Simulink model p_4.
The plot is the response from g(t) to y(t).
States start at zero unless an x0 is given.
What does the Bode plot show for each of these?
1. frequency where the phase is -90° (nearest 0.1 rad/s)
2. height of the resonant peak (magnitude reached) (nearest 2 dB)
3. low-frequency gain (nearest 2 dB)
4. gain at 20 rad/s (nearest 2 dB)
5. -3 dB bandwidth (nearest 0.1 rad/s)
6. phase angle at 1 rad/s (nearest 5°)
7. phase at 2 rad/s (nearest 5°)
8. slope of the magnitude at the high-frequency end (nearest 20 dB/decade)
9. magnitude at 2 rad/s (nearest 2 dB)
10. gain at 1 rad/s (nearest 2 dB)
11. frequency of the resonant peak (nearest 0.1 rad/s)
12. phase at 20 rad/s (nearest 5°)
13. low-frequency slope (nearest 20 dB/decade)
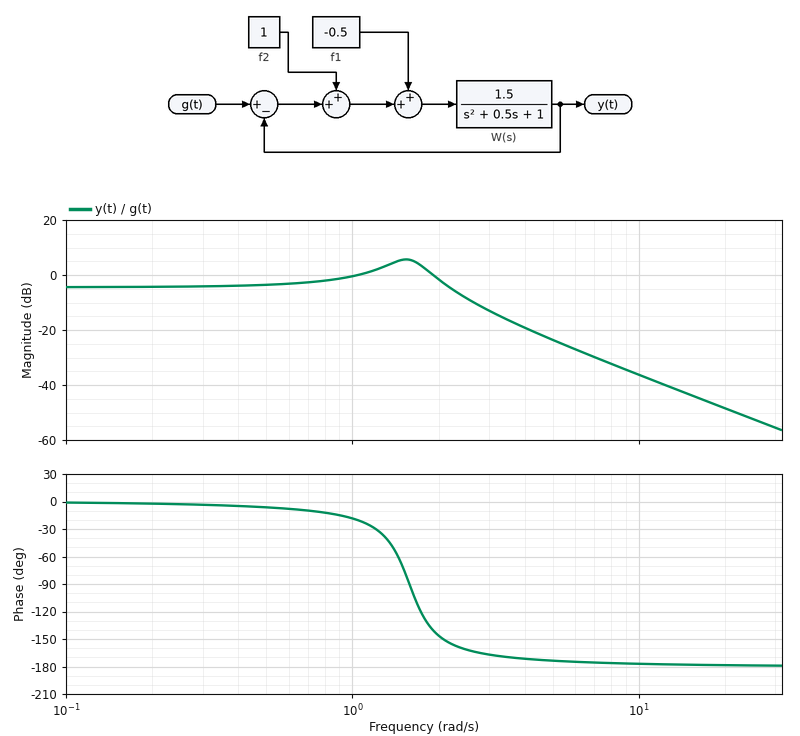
1.6 rad/s
6 dB
-4 dB
-48 dB
2.4 rad/s
-20°
-145°
-40 dB/decade
-2 dB
0 dB
1.5 rad/s
-180°
0 dB/decade
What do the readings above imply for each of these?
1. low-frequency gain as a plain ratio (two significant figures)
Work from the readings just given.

0.63
